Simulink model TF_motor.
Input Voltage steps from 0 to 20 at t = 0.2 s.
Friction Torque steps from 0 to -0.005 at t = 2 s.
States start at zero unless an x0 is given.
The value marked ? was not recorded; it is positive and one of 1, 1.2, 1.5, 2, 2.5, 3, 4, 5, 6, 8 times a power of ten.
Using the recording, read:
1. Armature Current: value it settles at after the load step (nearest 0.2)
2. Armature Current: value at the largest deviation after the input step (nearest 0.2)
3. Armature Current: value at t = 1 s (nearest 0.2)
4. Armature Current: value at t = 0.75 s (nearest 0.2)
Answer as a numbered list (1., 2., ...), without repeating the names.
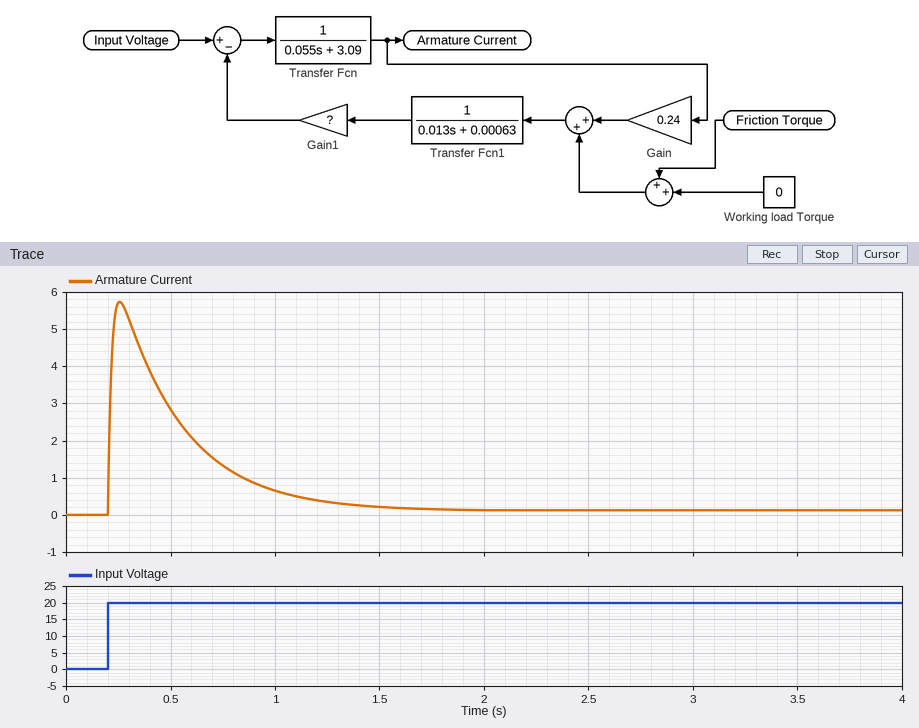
1. 0.2
2. 5.8
3. 0.6
4. 1.4
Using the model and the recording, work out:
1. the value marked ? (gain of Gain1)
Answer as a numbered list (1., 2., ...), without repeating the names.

1. 0.5
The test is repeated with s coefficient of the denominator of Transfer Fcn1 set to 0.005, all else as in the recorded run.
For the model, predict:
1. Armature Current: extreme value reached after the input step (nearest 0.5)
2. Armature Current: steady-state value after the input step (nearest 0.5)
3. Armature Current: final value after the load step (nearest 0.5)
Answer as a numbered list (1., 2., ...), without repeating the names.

1. 5.0
2. 0.0
3. 0.0
